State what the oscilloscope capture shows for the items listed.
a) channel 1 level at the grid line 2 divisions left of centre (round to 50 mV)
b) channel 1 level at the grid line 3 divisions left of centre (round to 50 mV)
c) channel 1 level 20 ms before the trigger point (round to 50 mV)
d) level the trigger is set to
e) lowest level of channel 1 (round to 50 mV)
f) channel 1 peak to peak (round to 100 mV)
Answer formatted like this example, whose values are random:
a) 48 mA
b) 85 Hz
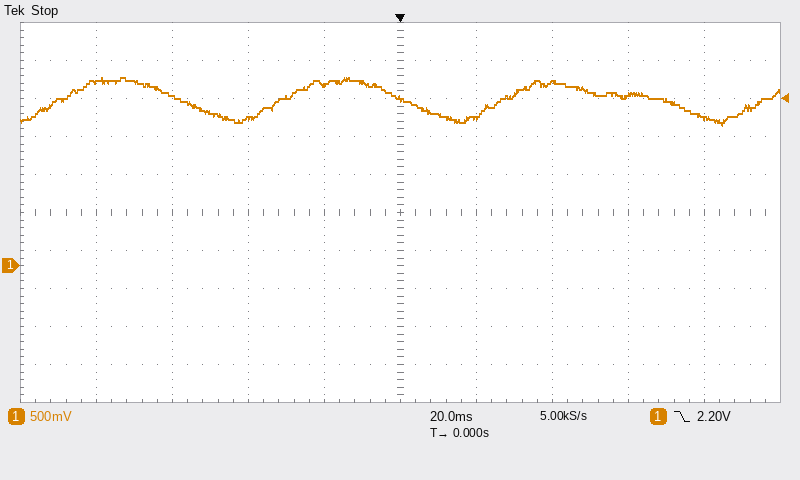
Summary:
a) 1.95 V
b) 2.25 V
c) 2.40 V
d) 2.20 V
e) 1.85 V
f) 600 mV
